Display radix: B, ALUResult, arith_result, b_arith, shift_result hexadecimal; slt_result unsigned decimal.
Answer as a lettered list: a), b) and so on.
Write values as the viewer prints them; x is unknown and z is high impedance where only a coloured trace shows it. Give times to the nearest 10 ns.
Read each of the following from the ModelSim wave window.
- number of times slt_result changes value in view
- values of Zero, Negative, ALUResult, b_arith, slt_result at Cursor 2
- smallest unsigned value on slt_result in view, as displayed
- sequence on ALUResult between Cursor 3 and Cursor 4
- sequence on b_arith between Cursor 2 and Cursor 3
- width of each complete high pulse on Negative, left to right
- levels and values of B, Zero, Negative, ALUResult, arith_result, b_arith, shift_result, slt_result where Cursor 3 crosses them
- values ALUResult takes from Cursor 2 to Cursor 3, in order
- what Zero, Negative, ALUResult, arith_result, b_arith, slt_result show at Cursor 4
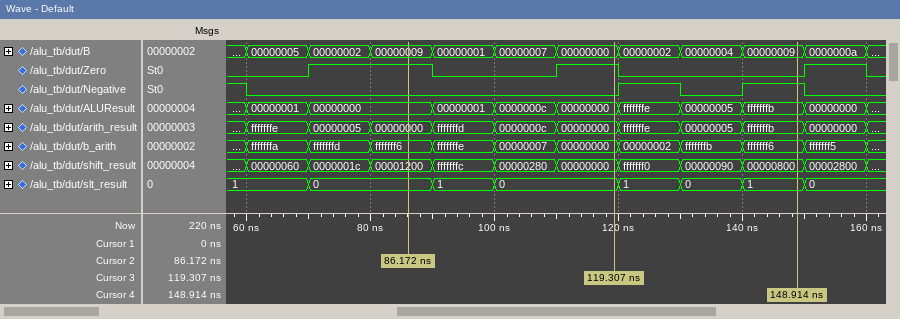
a) 7
b) Zero=1, Negative=0, ALUResult=00000000, b_arith=fffffff6, slt_result=0
c) 0
d) 00000000, fffffffe, 00000005, fffffffb
e) fffffff6, fffffffe, 00000007, 00000000
f) 10 ns, 10 ns
g) B=00000000, Zero=1, Negative=0, ALUResult=00000000, arith_result=00000000, b_arith=00000000, shift_result=00000000, slt_result=0
h) 00000000, 00000001, 0000000c, 00000000
i) Zero=0, Negative=1, ALUResult=fffffffb, arith_result=fffffffb, b_arith=fffffff6, slt_result=1
